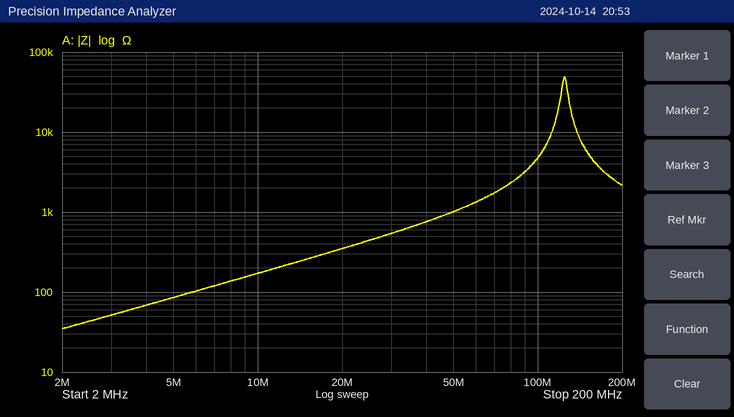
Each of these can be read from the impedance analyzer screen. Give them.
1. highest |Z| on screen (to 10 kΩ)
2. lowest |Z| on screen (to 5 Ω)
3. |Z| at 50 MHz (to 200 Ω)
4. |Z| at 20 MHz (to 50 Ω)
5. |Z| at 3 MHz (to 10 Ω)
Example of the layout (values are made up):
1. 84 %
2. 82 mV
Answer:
1. 50 kΩ
2. 35 Ω
3. 1.0 kΩ
4. 350 Ω
5. 50 Ω
